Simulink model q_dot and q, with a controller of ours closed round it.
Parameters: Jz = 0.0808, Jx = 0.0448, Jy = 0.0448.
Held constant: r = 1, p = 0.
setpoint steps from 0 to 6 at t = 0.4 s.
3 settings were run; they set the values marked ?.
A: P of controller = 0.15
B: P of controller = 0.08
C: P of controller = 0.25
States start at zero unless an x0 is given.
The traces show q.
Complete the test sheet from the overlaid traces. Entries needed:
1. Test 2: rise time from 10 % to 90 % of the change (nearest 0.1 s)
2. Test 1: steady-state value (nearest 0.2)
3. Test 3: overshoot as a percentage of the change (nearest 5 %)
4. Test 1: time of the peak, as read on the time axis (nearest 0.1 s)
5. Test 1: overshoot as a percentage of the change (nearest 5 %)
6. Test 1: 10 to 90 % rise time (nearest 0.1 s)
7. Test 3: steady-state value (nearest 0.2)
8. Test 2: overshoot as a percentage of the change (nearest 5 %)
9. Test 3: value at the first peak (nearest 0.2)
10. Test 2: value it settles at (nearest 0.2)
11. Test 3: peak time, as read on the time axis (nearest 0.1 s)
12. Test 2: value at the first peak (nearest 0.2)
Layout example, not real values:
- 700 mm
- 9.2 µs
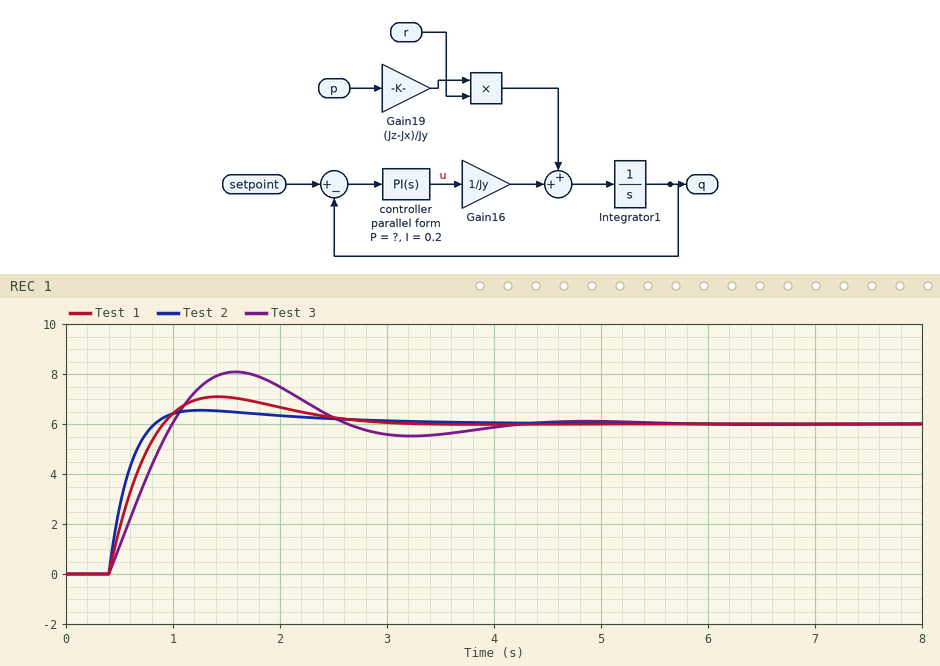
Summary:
- 0.3 s
- 6.0
- 35 %
- 1.4 s
- 20 %
- 0.4 s
- 6.0
- 10 %
- 8.0
- 6.0
- 1.6 s
- 6.6
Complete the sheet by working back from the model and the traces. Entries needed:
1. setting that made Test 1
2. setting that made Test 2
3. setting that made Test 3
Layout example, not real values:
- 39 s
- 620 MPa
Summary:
- A
- C
- B
